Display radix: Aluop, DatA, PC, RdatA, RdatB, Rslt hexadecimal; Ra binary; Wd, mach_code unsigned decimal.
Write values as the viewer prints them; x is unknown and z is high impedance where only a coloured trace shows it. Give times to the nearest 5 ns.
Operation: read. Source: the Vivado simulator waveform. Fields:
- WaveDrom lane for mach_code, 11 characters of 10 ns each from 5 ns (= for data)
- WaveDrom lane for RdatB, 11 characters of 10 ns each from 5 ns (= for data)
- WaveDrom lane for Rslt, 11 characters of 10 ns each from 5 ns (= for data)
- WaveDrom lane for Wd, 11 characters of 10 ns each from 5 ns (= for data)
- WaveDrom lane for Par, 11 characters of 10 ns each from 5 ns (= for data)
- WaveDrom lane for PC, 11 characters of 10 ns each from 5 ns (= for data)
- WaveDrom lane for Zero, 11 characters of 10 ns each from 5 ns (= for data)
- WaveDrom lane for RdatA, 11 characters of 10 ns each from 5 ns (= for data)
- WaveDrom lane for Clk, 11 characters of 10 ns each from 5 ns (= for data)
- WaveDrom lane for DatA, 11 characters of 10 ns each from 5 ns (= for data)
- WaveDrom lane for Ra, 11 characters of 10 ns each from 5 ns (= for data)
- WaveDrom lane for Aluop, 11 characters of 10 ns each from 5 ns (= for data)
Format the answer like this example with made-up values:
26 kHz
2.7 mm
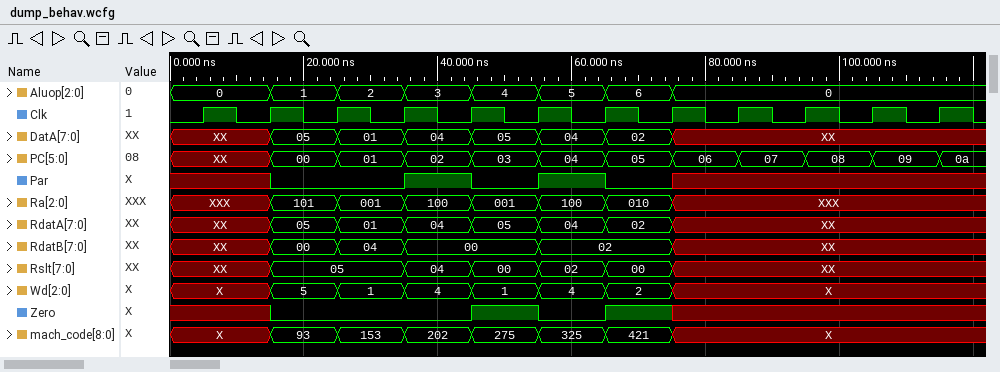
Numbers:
{name: 'mach_code', wave: 'x======x...', data: '93 153 202 275 325 421'}
{name: 'RdatB', wave: 'x===.=.x...', data: '00 04 00 02'}
{name: 'Rslt', wave: 'x=.====x...', data: '05 04 00 02 00'}
{name: 'Wd', wave: 'x======x...', data: '5 1 4 1 4 2'}
{name: 'Par', wave: 'x0.1010x...'}
{name: 'PC', wave: 'x==========', data: '00 01 02 03 04 05 06 07 08 09'}
{name: 'Zero', wave: 'x0..101x...'}
{name: 'RdatA', wave: 'x======x...', data: '05 01 04 05 04 02'}
{name: 'Clk', wave: 'p..........'}
{name: 'DatA', wave: 'x======x...', data: '05 01 04 05 04 02'}
{name: 'Ra', wave: 'x======x...', data: '101 001 100 001 100 010'}
{name: 'Aluop', wave: '========...', data: '0 1 2 3 4 5 6 0'}
